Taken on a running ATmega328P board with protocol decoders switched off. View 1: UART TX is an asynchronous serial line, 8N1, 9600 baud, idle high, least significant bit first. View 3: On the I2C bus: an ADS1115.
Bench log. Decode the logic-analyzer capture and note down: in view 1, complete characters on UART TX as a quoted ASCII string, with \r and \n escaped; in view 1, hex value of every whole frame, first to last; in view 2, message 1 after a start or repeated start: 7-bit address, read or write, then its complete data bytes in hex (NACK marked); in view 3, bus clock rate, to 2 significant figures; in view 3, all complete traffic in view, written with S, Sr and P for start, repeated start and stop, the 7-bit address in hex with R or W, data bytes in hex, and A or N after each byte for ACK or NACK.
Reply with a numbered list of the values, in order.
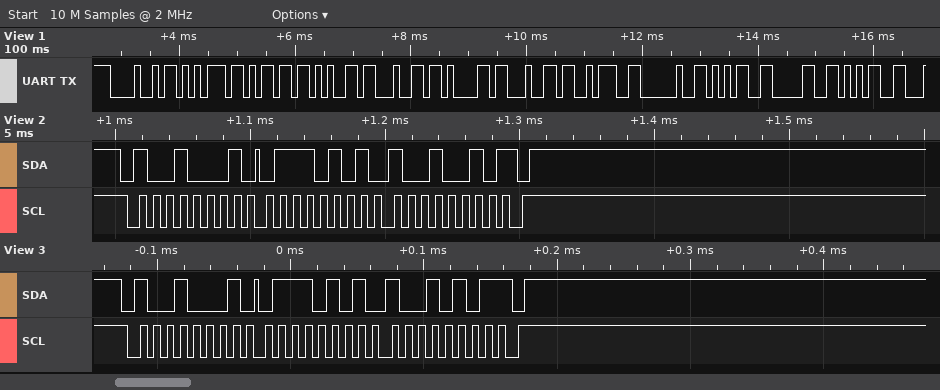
1. "Humedad: 505"
2. 48 75 6D 65 64 61 64 3A 20 35 30 35
3. 0x48 read: 75 92 NACK
4. 100 kHz
5. S 48R A 75 A 95 N P
